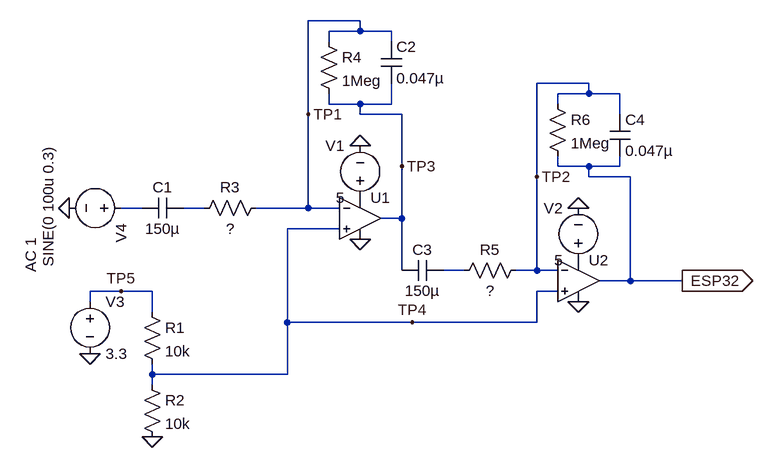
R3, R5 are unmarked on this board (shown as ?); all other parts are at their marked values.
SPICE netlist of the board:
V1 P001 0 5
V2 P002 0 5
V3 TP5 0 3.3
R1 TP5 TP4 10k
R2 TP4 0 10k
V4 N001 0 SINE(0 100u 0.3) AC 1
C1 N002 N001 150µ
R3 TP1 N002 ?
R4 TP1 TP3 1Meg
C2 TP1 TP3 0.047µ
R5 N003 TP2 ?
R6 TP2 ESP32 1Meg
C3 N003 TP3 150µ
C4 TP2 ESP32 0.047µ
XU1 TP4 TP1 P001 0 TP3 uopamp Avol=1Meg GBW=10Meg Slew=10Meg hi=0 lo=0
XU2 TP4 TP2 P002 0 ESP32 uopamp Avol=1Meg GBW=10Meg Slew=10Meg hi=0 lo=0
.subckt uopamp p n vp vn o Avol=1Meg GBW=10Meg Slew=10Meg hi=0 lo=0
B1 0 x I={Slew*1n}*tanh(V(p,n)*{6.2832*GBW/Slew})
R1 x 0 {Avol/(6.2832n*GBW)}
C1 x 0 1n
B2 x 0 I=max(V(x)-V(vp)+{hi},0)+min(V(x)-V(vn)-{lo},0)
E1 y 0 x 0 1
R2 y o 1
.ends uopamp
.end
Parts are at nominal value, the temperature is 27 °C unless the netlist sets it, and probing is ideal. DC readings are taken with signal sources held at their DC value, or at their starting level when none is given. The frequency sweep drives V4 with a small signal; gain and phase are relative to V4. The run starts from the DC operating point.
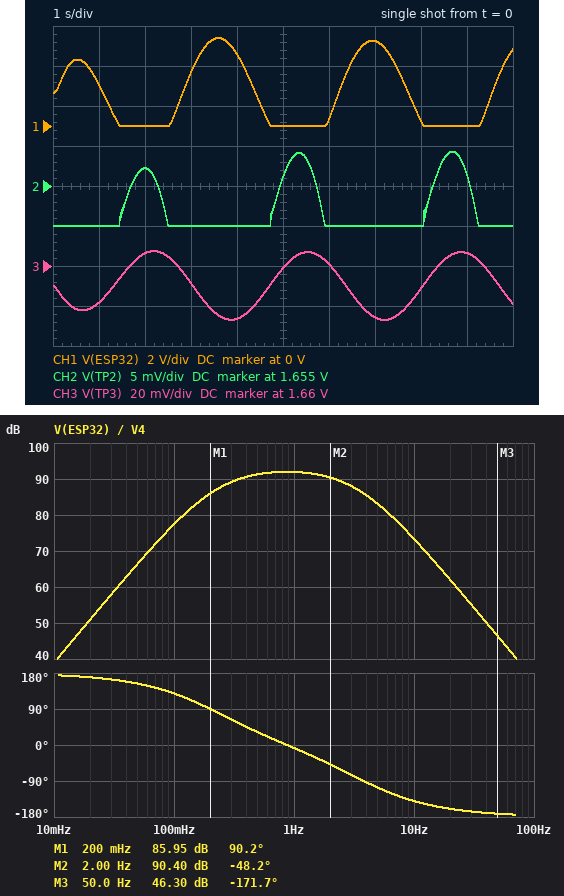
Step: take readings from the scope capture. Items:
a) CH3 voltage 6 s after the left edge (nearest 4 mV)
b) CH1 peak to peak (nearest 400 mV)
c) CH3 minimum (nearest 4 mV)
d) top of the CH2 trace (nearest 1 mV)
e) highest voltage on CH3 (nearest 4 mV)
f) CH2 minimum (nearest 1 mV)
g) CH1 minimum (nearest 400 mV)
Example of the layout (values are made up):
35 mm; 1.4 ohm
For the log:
1.660 V; 4.4 V; 1.632 V; 1.659 V; 1.668 V; 1.650 V; 0 V
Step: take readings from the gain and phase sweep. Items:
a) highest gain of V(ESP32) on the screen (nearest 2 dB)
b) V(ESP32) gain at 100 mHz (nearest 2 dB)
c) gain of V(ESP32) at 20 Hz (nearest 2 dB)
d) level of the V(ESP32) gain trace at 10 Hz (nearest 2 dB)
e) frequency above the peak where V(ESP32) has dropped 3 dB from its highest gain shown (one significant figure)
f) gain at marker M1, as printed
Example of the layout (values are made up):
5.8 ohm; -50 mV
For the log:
92 dB; 78 dB; 62 dB; 74 dB; 3 Hz; 85.95 dB
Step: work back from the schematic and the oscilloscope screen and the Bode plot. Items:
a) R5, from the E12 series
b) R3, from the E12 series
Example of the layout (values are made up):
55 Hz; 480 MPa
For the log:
4.7 kΩ; 4.7 kΩ
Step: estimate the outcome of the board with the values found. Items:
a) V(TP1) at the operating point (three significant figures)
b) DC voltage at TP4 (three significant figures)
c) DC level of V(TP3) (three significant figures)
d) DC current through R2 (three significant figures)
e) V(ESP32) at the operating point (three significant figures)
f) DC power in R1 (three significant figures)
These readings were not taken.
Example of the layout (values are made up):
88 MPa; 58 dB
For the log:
1.65 V; 1.65 V; 1.65 V; 165 µA; 1.65 V; 272 µW
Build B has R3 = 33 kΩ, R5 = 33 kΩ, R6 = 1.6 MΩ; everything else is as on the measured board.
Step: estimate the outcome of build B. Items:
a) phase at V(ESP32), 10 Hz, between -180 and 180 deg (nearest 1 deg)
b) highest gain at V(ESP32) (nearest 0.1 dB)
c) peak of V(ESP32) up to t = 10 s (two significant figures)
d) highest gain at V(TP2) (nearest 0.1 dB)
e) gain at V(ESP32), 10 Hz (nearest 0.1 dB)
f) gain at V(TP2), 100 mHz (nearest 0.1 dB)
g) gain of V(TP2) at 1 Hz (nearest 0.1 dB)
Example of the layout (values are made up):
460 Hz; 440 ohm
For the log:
-149 deg; 63.1 dB; 1.8 V; -56.9 dB; 39.8 dB; -57.5 dB; -57.9 dB
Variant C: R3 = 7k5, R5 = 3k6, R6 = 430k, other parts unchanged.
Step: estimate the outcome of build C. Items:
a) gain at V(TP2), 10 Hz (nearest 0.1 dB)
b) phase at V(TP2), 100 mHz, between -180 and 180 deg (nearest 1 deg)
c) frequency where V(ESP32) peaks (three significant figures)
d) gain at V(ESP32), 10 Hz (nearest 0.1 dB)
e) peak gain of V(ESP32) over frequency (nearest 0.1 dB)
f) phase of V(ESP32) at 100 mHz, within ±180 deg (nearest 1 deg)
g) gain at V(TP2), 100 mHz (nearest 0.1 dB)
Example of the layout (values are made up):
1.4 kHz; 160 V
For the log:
-47.0 dB; -56 deg; 1.01 Hz; 70.0 dB; 83.2 dB; 124 deg; -50.6 dB
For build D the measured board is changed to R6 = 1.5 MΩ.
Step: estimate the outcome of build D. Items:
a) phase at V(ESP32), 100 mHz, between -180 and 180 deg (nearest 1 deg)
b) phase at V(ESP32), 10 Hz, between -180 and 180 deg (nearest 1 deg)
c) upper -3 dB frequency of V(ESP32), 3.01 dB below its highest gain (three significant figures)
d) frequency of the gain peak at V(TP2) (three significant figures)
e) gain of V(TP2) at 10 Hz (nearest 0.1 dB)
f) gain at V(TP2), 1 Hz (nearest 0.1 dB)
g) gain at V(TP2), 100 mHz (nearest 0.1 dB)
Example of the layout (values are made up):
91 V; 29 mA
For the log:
128 deg; -146 deg; 2.17 Hz; 785 mHz; -43.4 dB; -24.9 dB; -39.1 dB
